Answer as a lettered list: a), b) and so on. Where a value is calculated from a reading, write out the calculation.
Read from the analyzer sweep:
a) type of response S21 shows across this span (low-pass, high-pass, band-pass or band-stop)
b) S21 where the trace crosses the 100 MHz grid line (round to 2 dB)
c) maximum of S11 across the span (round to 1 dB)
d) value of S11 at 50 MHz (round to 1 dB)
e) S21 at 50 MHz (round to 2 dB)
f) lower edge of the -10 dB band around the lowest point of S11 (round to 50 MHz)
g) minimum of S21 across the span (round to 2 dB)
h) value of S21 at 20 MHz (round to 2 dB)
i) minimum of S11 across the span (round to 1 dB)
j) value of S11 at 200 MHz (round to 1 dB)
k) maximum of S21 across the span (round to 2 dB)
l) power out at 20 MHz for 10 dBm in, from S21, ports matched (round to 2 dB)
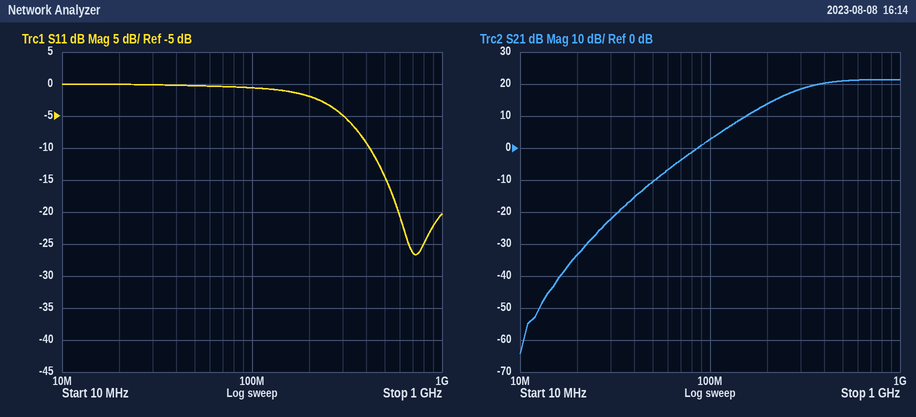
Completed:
a) high-pass
b) 2 dB
c) 0 dB
d) 0 dB
e) -10 dB
f) 400 MHz
g) -64 dB
h) -34 dB
i) -27 dB
j) -2 dB
k) 22 dB
l) 10 dBm + (-34 dB) = -24 dBm
